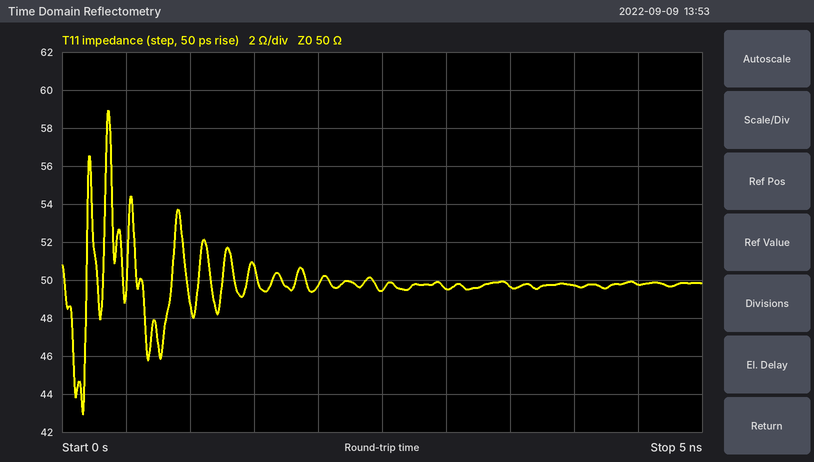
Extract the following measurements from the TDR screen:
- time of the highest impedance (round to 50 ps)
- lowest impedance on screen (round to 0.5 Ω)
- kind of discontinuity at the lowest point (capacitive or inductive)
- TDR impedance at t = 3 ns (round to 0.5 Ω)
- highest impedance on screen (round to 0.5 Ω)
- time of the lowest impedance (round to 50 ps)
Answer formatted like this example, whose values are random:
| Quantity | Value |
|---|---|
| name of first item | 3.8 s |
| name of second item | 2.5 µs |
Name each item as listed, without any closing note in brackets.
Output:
| Quantity | Value |
|---|---|
| time of the highest impedance | 350 ps |
| lowest impedance on screen | 43.0 Ω |
| kind of discontinuity at the lowest point | capacitive |
| TDR impedance at t = 3 ns | 49.5 Ω |
| highest impedance on screen | 59.0 Ω |
| time of the lowest impedance | 150 ps |
